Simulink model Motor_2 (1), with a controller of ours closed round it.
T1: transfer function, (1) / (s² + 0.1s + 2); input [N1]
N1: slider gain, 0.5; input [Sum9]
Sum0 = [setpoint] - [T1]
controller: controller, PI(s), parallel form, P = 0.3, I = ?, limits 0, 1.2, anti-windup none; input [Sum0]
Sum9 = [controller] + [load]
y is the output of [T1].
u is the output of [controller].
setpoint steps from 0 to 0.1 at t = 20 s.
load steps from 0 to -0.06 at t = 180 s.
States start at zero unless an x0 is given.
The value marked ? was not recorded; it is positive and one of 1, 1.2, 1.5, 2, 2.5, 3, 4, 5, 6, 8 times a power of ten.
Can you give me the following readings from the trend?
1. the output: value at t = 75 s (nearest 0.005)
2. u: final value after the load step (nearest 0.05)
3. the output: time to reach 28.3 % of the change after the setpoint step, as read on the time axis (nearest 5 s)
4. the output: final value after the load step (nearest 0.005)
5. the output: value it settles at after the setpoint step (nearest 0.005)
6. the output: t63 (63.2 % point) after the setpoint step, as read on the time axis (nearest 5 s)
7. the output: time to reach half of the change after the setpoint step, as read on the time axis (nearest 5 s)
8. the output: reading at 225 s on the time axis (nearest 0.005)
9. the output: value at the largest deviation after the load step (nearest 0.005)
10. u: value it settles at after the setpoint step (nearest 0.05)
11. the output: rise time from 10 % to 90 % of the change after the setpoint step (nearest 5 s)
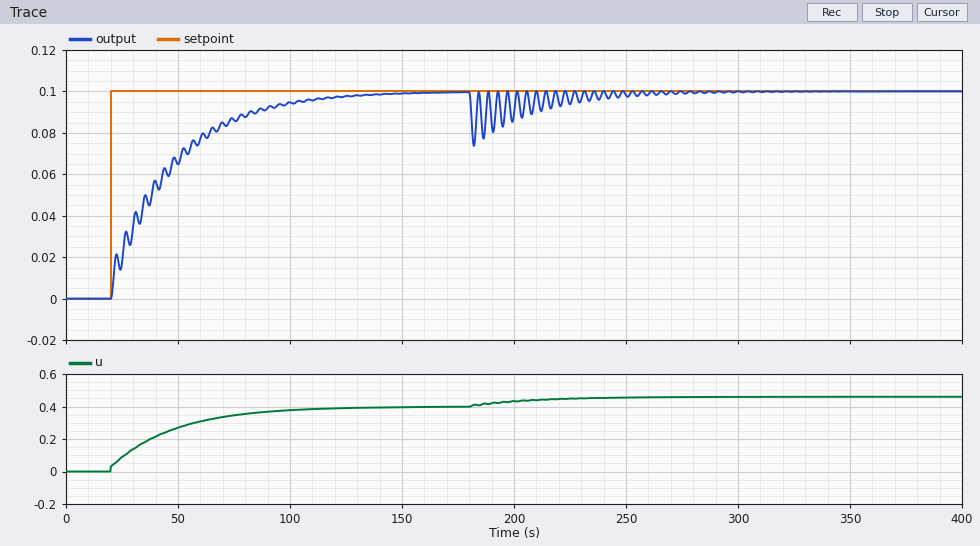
0.085
0.45
25 s
0.100
0.100
45 s
40 s
0.095
0.075
0.40
60 s
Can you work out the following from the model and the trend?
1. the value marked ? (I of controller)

0.15
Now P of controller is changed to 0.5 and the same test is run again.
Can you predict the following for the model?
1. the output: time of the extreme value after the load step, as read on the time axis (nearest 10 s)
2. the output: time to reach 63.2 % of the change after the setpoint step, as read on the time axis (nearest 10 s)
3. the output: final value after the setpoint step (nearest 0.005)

180 s
40 s
0.100
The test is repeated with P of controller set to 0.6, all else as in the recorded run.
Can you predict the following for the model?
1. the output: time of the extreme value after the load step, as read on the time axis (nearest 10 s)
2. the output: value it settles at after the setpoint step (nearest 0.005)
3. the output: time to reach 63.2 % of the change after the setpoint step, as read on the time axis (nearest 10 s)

180 s
0.100
40 s
